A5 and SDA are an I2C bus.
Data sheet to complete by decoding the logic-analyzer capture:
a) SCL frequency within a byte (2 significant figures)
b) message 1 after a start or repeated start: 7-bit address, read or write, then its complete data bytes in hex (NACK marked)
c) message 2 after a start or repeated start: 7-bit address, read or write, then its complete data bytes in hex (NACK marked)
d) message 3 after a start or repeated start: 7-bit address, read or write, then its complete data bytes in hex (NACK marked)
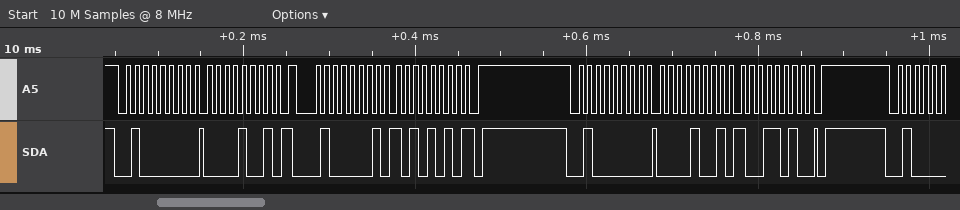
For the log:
100 kHz
0x20 write: 09
0x20 read: AA NACK
0x20 write: 09 9A
